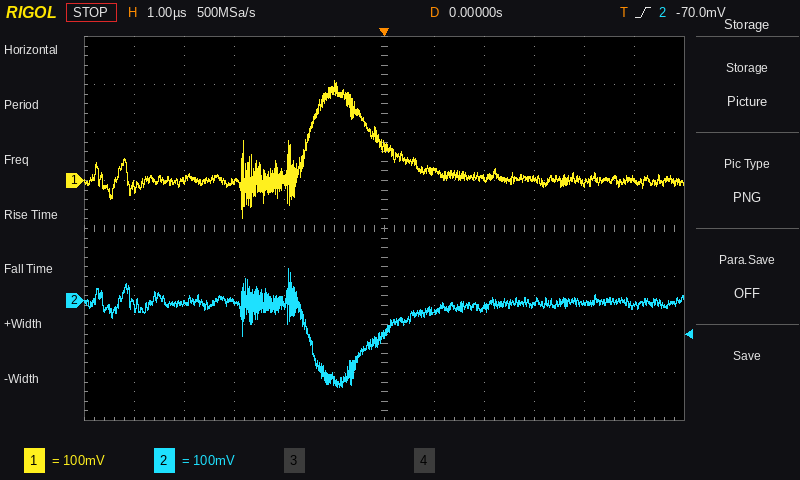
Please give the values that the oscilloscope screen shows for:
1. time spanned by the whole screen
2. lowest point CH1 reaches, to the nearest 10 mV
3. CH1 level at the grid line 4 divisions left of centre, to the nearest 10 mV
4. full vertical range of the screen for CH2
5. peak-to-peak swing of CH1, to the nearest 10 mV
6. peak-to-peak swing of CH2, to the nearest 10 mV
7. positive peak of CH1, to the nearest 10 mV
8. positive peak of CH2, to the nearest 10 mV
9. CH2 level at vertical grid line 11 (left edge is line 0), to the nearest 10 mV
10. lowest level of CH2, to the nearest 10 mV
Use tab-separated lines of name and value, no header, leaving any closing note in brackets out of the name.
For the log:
time spanned by the whole screen	12 µs
lowest point CH1 reaches, to the nearest 10 mV	-80 mV
CH1 level at the grid line 4 divisions left of centre, to the nearest 10 mV	0 mV
full vertical range of the screen for CH2	800 mV
peak-to-peak swing of CH1, to the nearest 10 mV	290 mV
peak-to-peak swing of CH2, to the nearest 10 mV	250 mV
positive peak of CH1, to the nearest 10 mV	210 mV
positive peak of CH2, to the nearest 10 mV	70 mV
CH2 level at vertical grid line 11 (left edge is line 0), to the nearest 10 mV	-10 mV
lowest level of CH2, to the nearest 10 mV	-180 mV
